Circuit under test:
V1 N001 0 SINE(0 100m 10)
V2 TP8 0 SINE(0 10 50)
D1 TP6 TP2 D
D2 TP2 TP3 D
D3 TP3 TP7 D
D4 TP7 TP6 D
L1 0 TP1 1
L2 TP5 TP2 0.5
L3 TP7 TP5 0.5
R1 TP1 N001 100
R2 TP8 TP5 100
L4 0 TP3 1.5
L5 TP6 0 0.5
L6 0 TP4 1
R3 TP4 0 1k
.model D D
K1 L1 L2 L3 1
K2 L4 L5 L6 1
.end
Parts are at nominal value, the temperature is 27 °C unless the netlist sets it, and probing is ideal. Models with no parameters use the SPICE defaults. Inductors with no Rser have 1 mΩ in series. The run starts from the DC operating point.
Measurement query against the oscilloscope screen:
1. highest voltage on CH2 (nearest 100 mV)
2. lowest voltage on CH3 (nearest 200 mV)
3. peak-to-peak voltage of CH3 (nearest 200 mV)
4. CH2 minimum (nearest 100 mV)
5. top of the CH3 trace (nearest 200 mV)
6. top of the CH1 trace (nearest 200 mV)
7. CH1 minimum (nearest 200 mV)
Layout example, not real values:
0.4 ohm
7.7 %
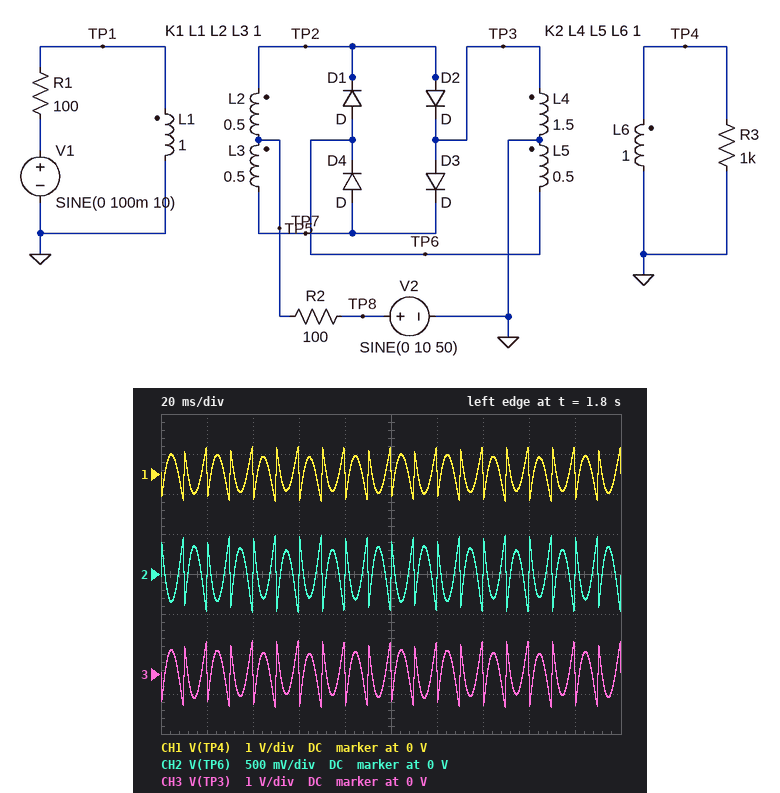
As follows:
500 mV
-800 mV
1.6 V
-500 mV
800 mV
600 mV
-600 mV
